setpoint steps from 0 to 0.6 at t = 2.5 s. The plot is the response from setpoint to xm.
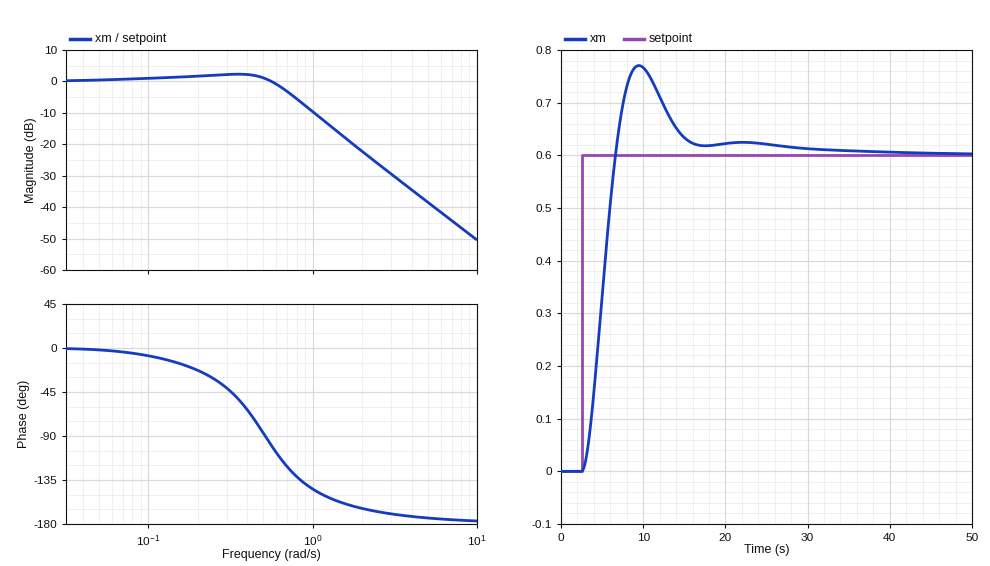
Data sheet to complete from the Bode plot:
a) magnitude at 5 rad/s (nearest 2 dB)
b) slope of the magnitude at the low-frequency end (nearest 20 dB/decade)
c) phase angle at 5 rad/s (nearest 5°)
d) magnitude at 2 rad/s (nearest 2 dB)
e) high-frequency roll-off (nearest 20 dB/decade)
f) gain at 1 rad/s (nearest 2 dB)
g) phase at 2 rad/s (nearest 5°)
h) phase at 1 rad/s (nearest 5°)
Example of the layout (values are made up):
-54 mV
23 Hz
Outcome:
-38 dB
0 dB/decade
-175°
-22 dB
-40 dB/decade
-10 dB
-165°
-145°
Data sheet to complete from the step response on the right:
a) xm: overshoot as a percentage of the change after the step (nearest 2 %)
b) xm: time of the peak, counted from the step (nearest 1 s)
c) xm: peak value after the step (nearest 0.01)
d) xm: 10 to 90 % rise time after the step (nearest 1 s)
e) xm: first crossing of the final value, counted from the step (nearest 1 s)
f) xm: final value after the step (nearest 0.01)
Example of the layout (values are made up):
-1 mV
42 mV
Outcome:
28 %
7 s
0.77
3 s
4 s
0.60
